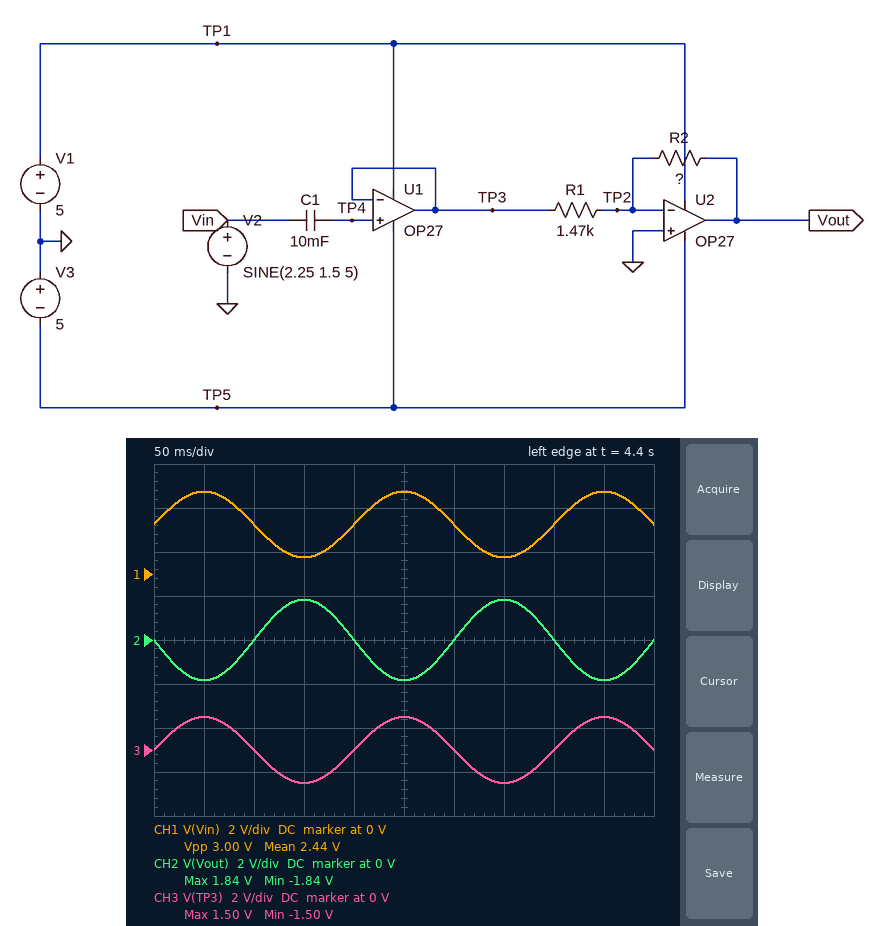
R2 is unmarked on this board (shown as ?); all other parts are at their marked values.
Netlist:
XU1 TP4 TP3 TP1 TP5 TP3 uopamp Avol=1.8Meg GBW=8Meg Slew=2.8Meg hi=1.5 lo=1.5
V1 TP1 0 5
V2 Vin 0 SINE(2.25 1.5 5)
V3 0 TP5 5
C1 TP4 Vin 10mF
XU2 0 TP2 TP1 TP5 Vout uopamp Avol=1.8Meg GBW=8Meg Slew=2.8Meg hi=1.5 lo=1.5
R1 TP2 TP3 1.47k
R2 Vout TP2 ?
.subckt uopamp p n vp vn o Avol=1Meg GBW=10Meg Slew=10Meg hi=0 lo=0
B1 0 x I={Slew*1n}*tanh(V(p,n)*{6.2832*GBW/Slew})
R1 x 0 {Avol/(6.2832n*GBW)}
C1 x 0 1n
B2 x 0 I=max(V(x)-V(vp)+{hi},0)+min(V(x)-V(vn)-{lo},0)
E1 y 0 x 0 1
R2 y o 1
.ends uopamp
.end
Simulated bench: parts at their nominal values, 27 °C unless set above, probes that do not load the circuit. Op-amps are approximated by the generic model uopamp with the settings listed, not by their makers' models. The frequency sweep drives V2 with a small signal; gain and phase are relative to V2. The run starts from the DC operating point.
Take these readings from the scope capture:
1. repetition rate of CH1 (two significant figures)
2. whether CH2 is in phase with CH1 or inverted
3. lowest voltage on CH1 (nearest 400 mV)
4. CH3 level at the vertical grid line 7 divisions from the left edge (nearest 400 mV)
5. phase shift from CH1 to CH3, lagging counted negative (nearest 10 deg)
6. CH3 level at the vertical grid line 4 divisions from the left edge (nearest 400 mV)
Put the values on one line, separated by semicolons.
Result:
5.0 Hz; inverted; 800 mV; -1.6 V; 0 deg; 0 V
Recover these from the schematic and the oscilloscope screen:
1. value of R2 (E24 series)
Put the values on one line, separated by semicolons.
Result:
1.8 kΩ
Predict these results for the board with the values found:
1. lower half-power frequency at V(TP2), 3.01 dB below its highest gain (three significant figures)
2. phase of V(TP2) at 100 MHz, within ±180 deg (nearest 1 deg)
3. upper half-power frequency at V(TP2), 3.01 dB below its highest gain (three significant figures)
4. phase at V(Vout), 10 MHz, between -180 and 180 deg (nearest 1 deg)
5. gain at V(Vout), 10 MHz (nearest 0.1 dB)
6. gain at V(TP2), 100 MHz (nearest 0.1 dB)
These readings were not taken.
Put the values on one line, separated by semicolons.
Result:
2.10 MHz; -83 deg; 13.7 MHz; 58 deg; -11.7 dB; -27.2 dB
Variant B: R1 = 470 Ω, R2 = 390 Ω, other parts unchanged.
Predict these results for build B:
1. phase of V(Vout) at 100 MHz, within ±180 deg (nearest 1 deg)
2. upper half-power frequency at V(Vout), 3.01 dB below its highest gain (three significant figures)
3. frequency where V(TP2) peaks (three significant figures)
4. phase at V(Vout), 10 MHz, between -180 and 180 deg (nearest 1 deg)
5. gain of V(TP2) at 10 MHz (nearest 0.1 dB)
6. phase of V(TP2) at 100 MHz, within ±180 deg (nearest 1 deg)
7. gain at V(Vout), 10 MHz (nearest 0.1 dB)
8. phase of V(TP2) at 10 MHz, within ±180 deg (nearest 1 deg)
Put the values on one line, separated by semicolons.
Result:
5 deg; 3.57 MHz; 5.91 MHz; 62 deg; -11.7 dB; -83 deg; -13.7 dB; -28 deg
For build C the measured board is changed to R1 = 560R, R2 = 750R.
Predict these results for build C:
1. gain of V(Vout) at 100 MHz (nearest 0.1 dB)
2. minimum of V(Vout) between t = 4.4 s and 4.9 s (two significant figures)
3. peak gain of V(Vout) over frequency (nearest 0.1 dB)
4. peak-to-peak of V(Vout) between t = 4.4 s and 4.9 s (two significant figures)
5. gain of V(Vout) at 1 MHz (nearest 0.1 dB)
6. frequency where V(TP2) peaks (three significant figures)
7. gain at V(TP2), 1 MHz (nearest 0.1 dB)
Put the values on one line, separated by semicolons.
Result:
-48.8 dB; -2.0 V; 2.5 dB; 4.0 V; 2.1 dB; 5.23 MHz; -15.9 dB
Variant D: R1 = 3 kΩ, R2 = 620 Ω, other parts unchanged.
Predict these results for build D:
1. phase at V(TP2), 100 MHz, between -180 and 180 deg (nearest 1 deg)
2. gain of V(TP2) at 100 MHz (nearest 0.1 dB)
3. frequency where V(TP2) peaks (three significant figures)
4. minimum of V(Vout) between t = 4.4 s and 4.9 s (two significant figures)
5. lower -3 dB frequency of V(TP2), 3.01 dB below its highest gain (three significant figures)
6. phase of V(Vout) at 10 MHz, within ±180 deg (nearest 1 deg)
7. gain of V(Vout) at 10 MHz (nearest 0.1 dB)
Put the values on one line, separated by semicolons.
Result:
-82 deg; -37.3 dB; 7.28 MHz; -310 mV; 3.01 MHz; 72 deg; -22.9 dB
